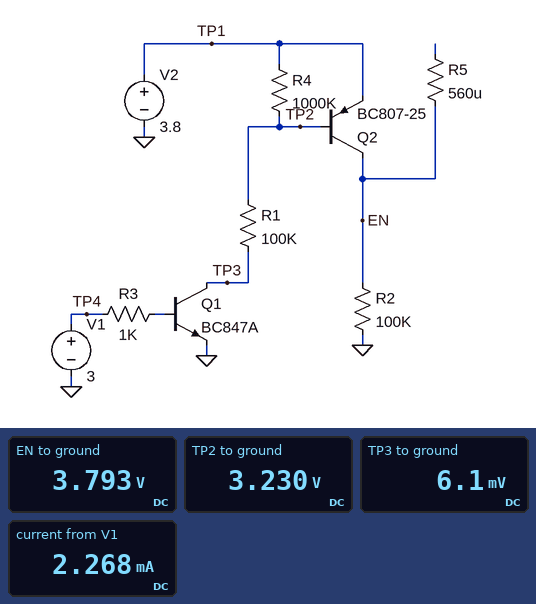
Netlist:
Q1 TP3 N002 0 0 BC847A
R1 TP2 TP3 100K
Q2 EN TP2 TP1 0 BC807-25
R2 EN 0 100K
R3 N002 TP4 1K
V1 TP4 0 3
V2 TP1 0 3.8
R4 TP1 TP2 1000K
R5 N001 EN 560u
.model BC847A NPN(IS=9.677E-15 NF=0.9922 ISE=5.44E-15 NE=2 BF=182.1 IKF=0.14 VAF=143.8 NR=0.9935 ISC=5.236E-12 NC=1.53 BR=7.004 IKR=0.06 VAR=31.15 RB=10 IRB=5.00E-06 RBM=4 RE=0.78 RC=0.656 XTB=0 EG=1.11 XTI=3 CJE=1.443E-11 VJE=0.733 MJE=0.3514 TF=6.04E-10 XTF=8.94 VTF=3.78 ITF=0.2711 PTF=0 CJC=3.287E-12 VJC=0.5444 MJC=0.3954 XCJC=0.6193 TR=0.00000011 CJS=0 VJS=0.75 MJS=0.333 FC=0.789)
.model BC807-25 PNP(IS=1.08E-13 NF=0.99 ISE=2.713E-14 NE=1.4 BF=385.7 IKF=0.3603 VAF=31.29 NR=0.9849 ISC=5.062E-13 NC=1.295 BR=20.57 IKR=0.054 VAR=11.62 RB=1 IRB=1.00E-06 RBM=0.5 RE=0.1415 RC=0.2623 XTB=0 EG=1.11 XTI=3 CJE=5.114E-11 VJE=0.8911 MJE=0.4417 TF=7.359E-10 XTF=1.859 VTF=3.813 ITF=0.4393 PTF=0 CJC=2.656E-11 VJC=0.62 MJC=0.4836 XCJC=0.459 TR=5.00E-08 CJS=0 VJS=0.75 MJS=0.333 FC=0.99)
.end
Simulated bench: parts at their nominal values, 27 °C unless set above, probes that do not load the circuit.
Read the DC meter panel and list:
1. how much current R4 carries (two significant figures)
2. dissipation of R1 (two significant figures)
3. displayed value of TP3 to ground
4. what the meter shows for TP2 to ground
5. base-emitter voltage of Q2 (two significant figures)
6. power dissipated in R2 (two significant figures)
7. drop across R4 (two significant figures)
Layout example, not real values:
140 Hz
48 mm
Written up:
570 nA
100 µW
6.1 mV
3.230 V
-570 mV
140 µW
570 mV
